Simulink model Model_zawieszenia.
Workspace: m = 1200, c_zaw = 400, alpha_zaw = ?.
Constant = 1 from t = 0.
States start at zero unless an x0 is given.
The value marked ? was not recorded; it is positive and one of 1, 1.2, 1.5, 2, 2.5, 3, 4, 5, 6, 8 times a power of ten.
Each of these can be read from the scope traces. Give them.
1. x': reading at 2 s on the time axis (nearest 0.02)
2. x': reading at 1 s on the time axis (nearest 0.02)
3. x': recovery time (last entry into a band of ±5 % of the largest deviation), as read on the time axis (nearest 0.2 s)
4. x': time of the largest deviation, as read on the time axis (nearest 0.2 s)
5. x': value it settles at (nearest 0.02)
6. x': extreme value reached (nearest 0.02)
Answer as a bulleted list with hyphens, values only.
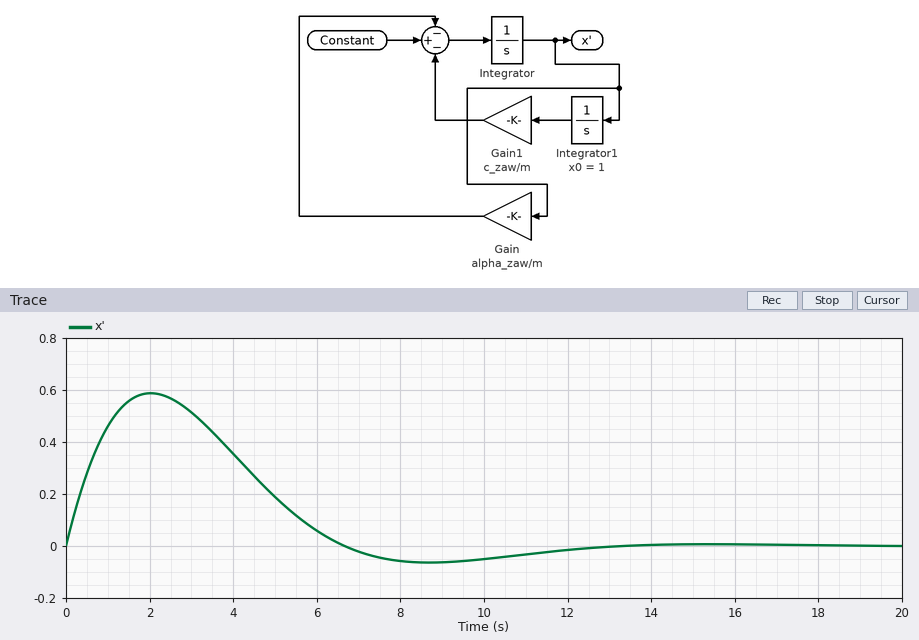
- 0.58
- 0.46
- 11.2 s
- 2.0 s
- 0.00
- 0.58
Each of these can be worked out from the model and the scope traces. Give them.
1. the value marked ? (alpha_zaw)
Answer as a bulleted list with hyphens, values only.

- 800
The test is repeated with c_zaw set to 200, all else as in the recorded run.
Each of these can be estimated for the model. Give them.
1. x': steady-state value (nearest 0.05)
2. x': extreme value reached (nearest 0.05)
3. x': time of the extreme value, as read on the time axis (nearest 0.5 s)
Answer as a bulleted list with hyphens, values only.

- 0.00
- 0.85
- 2.5 s
